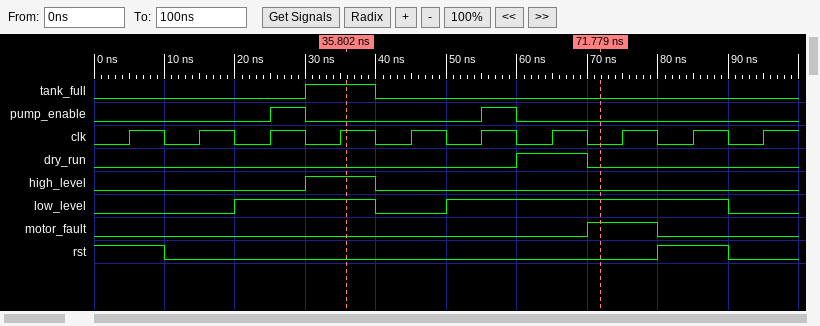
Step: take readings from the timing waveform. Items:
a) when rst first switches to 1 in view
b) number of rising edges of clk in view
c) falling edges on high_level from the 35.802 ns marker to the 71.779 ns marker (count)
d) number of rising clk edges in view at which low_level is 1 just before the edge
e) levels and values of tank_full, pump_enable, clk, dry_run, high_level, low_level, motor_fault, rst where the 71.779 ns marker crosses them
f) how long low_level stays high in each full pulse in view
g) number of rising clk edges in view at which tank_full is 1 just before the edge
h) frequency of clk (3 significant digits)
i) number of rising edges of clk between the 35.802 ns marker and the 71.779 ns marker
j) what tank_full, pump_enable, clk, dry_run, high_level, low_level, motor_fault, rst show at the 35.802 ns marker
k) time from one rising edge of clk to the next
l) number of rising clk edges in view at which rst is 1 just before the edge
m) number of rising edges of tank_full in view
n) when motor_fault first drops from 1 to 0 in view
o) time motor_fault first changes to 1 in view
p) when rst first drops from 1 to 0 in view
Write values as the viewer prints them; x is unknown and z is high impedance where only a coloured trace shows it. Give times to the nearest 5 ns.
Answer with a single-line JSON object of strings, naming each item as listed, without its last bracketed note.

{"when rst first switches to 1 in view": "80 ns", "number of rising edges of clk in view": "10", "falling edges on high_level from the 35.802 ns marker to the 71.779 ns marker": "1", "number of rising clk edges in view at which low_level is 1 just before the edge": "6", "levels and values of tank_full, pump_enable, clk, dry_run, high_level, low_level, motor_fault, rst where the 71.779 ns marker crosses them": "tank_full=0, pump_enable=0, clk=0, dry_run=0, high_level=0, low_level=1, motor_fault=1, rst=0", "how long low_level stays high in each full pulse in view": "20 ns, 40 ns", "number of rising clk edges in view at which tank_full is 1 just before the edge": "1", "frequency of clk": "100 MHz", "number of rising edges of clk between the 35.802 ns marker and the 71.779 ns marker": "3", "what tank_full, pump_enable, clk, dry_run, high_level, low_level, motor_fault, rst show at the 35.802 ns marker": "tank_full=1, pump_enable=0, clk=1, dry_run=0, high_level=1, low_level=1, motor_fault=0, rst=0", "time from one rising edge of clk to the next": "10 ns", "number of rising clk edges in view at which rst is 1 just before the edge": "2", "number of rising edges of tank_full in view": "1", "when motor_fault first drops from 1 to 0 in view": "80 ns", "time motor_fault first changes to 1 in view": "70 ns", "when rst first drops from 1 to 0 in view": "10 ns"}
